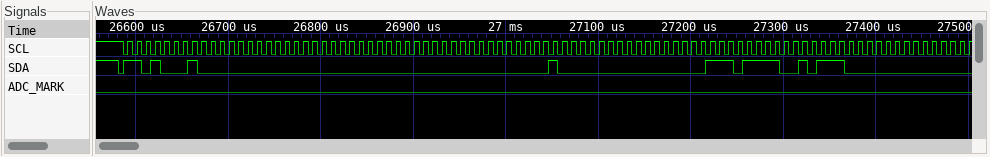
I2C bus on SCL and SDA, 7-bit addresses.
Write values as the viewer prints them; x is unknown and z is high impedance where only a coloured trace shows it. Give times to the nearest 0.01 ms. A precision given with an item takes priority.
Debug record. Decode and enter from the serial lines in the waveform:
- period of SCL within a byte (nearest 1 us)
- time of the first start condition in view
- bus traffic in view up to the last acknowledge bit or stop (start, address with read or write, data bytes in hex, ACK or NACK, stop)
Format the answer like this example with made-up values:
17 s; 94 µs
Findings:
10 us; 26.58 ms; start, address 68 read ACK, 00 ACK, 00 ACK, 00 ACK, 00 ACK, 40 ACK, 00 ACK, EF ACK, 5C ACK, 00 ACK
